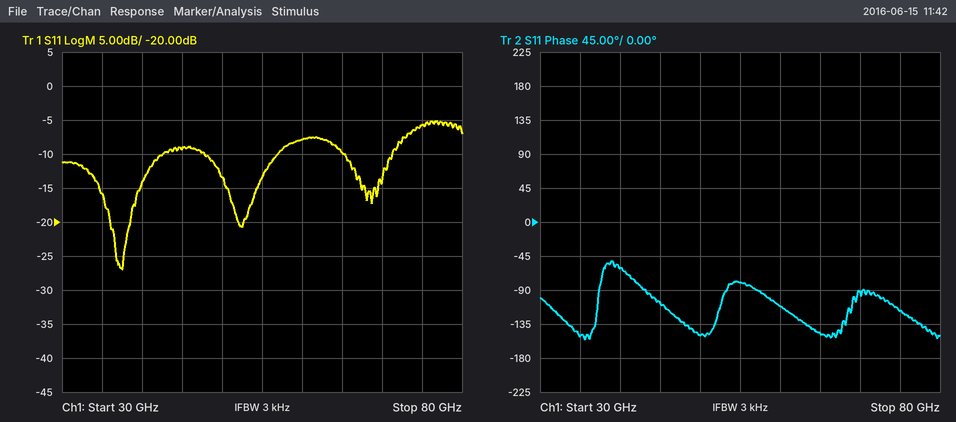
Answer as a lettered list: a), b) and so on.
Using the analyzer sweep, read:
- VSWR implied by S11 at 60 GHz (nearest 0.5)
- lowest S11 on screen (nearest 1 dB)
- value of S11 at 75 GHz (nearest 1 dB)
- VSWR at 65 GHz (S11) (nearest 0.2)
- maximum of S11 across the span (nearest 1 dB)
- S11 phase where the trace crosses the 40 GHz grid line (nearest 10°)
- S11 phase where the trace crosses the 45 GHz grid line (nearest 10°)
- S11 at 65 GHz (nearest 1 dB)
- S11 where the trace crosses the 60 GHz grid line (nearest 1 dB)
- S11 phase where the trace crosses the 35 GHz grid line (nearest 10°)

a) 2.5
b) -27 dB
c) -6 dB
d) 2.0
e) -5 dB
f) -60°
g) -110°
h) -10 dB
i) -8 dB
j) -150°
